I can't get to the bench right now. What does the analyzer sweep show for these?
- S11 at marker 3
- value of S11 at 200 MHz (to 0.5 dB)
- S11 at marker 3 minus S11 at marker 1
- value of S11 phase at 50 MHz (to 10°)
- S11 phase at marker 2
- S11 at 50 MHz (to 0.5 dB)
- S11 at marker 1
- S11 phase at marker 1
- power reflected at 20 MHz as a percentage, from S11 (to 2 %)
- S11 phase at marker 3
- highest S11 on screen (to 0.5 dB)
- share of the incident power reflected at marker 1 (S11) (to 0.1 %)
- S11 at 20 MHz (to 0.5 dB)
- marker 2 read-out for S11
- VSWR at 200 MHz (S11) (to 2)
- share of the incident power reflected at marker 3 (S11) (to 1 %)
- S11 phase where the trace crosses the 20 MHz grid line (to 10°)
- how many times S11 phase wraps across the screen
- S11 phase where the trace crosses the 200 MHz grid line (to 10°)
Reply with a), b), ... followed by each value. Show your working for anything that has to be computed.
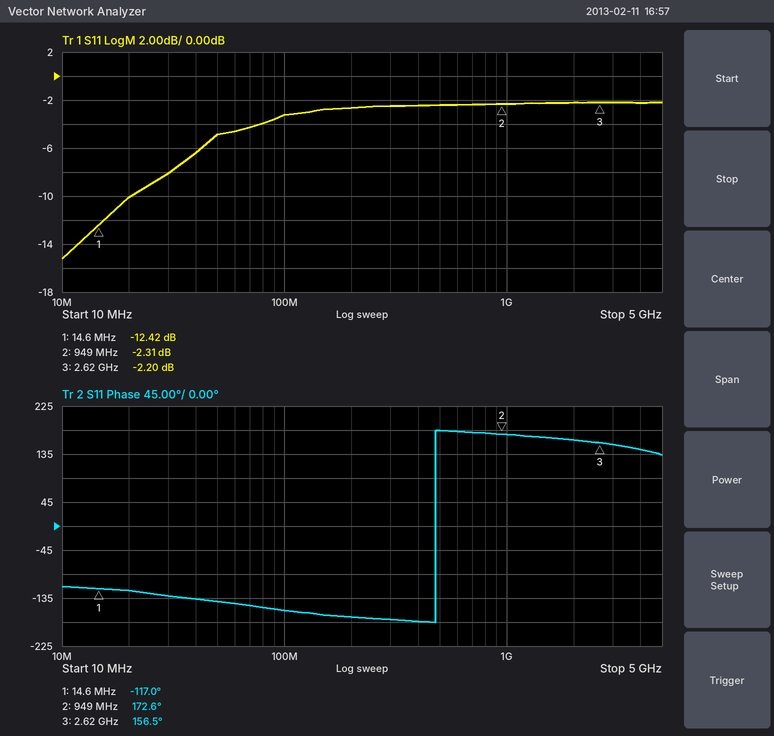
a) -2.20 dB
b) -2.5 dB
c) -2.2 − (-12.42) = 10.22 dB
d) -140°
e) 172.6°
f) -5.0 dB
g) -12.42 dB
h) -117.0°
i) 10^(-10/10) ≈ 10 %
j) 156.5°
k) -2.0 dB
l) 10^(-12.42/10) ≈ 5.7 %
m) -10.0 dB
n) -2.31 dB
o) |Γ| = 10^(-2.5/20) = 0.7499; VSWR = (1 + 0.7499)/(1 − 0.7499) ≈ 7.00, so 6 to the nearest 2
p) 10^(-2.2/10) ≈ 60 %
q) -120°
r) 1
s) -170°
